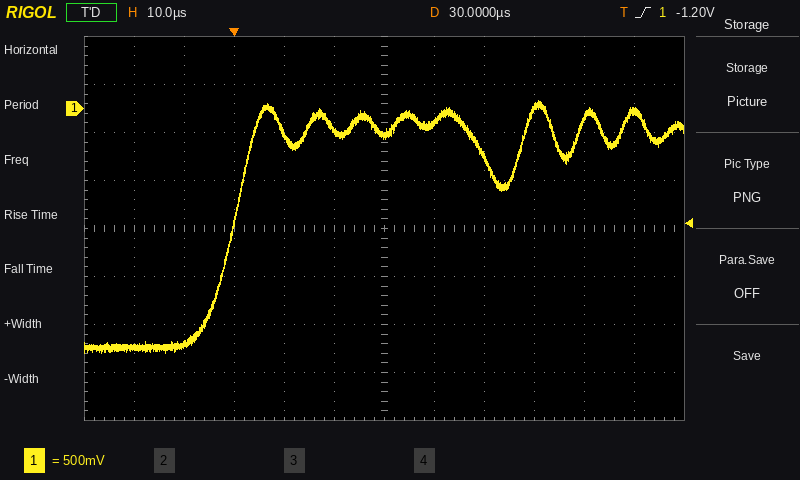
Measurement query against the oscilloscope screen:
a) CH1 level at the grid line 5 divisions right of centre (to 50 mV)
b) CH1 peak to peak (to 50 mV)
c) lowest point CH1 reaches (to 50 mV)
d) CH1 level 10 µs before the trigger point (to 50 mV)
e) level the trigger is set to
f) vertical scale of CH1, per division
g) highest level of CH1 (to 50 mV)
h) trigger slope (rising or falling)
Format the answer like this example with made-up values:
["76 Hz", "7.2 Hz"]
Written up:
["-50 mV", "2.65 V", "-2.55 V", "-2.45 V", "-1.20 V", "500 mV", "100 mV", "rising"]
